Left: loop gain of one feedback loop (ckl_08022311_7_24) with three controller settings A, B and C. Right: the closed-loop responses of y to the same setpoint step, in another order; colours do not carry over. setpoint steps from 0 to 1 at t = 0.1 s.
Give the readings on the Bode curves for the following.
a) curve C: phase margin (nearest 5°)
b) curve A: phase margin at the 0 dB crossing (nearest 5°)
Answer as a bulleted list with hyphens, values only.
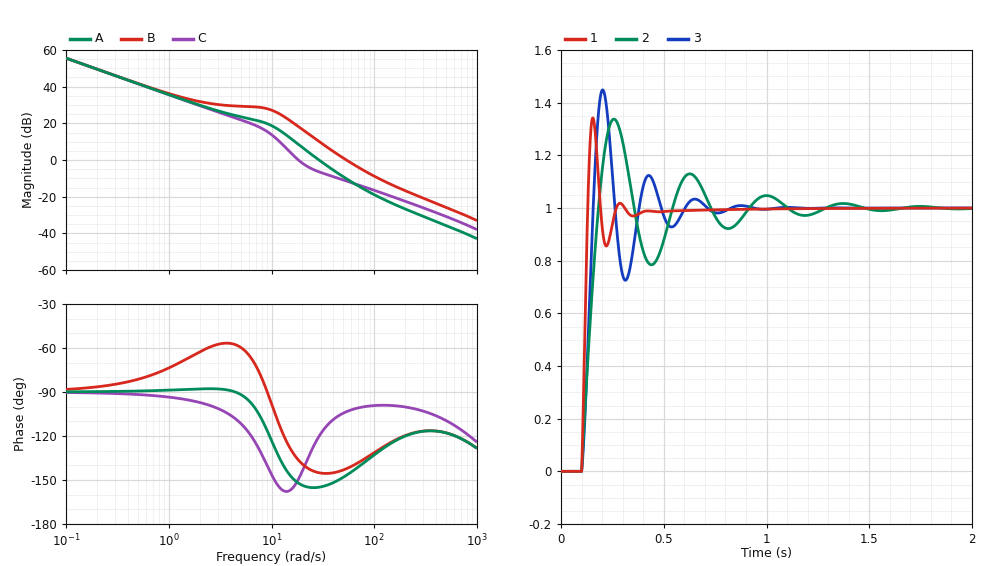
- 30°
- 25°
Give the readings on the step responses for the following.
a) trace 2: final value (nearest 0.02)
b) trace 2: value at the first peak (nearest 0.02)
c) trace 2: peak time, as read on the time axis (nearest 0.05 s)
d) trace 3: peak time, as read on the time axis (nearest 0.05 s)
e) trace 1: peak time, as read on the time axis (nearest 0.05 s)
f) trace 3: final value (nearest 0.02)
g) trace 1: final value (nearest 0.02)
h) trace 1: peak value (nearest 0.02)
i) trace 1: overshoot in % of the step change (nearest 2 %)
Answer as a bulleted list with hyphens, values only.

- 1.00
- 1.34
- 0.25 s
- 0.20 s
- 0.15 s
- 1.00
- 1.00
- 1.34
- 34 %
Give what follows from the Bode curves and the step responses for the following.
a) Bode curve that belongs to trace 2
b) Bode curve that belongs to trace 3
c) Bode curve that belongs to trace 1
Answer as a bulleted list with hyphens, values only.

- C
- A
- B
